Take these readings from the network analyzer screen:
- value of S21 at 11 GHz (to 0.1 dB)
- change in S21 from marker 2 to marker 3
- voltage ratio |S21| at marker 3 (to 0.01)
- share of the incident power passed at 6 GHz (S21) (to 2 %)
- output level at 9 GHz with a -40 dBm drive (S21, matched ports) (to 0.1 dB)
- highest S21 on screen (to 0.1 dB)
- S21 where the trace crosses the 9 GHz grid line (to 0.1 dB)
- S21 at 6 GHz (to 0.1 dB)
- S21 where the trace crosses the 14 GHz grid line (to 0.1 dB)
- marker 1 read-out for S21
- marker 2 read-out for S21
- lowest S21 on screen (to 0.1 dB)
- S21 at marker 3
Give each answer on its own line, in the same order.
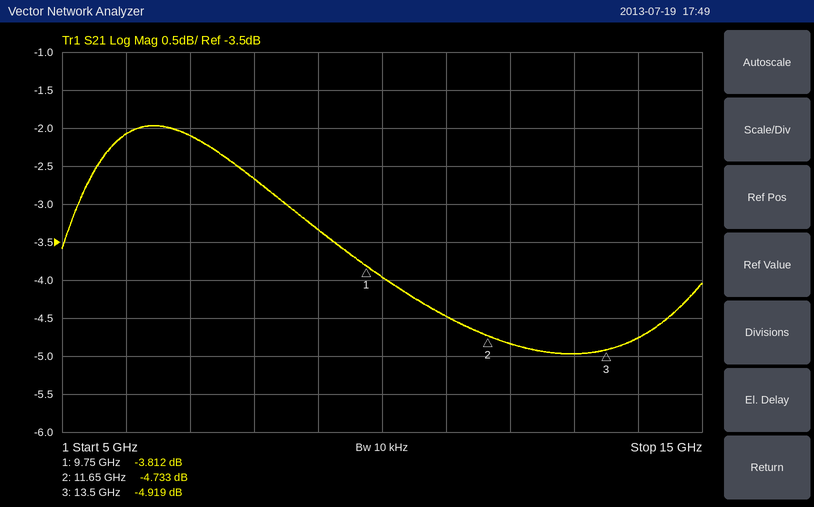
-4.5 dB
-0.186 dB
0.57
62 %
-43.3 dBm
-2.0 dB
-3.3 dB
-2.1 dB
-4.8 dB
-3.812 dB
-4.733 dB
-5.0 dB
-4.919 dB
